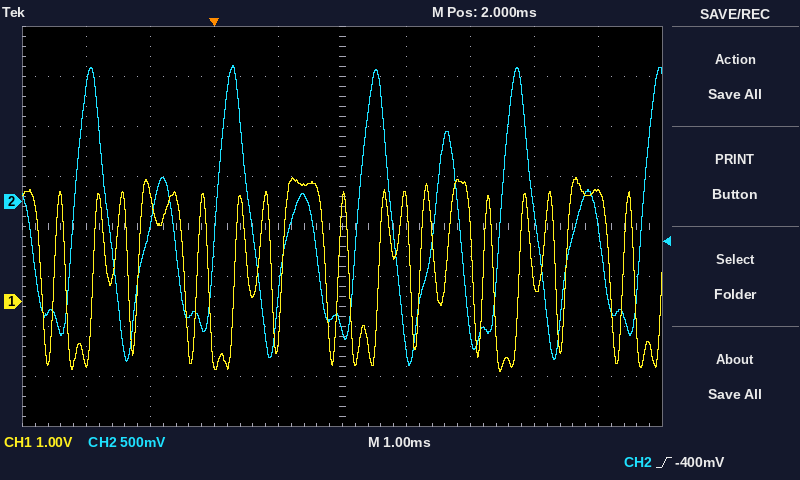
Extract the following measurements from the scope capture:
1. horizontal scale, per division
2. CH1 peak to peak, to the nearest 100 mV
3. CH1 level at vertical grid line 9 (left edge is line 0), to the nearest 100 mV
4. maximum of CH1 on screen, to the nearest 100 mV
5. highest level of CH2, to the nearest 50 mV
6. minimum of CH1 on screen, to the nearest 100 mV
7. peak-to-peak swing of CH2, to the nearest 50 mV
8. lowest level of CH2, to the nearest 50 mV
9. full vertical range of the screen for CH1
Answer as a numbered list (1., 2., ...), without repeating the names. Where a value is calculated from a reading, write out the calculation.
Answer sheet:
1. 1 ms
2. 2.5 V − (-1.4 V) = 3.9 V
3. 2.2 V
4. 2.5 V
5. 1.35 V
6. -1.4 V
7. 1.35 V − (-1.65 V) = 3.00 V
8. -1.65 V
9. 8 V
